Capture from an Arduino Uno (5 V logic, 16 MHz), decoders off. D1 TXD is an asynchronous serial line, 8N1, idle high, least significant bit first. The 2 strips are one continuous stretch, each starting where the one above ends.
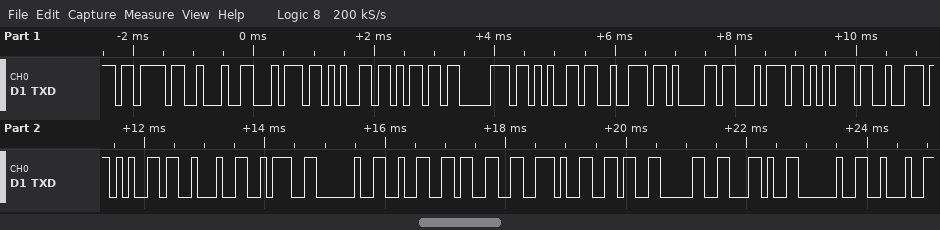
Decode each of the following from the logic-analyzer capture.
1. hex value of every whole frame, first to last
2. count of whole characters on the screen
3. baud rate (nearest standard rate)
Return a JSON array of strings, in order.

["0x7B 0x22 0x74 0x65 0x6D 0x70 0x65 0x72 0x61 0x74 0x75 0x72 0x65 0x22 0x3A 0x20 0x32 0x33 0x2E 0x36 0x30 0x2C 0x20 0x22", "24", "9600 baud"]
